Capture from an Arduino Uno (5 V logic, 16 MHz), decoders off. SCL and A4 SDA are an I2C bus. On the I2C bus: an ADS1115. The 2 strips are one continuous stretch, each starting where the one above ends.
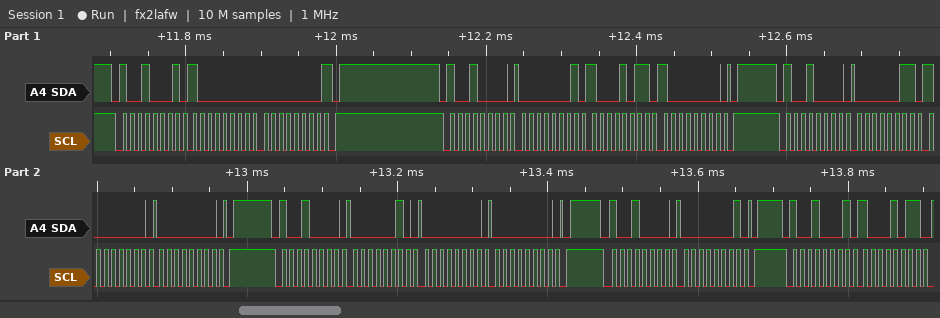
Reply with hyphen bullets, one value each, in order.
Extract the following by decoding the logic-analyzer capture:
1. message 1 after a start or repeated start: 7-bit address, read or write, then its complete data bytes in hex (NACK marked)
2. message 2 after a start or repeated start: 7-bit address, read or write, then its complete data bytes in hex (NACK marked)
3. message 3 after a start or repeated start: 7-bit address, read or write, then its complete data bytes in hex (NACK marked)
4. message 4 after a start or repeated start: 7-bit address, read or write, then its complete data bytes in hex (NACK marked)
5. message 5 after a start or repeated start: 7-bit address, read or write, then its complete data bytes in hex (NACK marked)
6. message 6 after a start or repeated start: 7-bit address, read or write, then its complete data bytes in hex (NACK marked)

- 0x48 read: 80 00 NACK
- 0x48 write: 01 8B 80
- 0x48 write: 03 80 00
- 0x48 write: 02 00 00
- 0x48 write: 01
- 0x48 read: 8B
